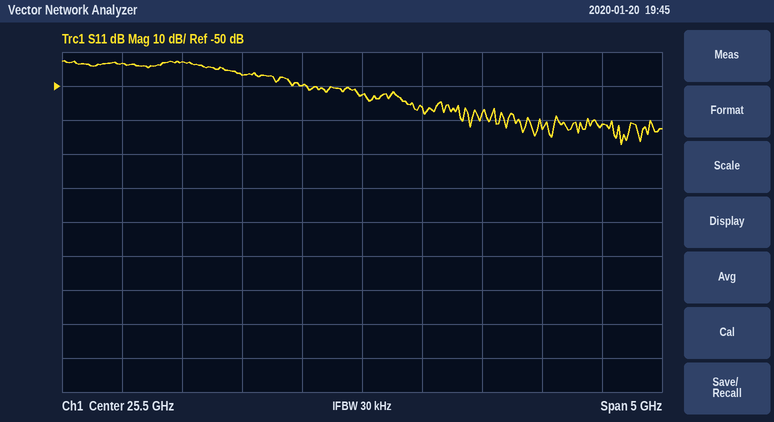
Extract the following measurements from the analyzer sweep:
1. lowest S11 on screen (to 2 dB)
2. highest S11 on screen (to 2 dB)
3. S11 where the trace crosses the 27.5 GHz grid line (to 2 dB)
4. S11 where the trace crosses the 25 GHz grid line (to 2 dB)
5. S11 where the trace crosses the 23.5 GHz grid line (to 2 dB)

-68 dB
-42 dB
-62 dB
-50 dB
-44 dB
